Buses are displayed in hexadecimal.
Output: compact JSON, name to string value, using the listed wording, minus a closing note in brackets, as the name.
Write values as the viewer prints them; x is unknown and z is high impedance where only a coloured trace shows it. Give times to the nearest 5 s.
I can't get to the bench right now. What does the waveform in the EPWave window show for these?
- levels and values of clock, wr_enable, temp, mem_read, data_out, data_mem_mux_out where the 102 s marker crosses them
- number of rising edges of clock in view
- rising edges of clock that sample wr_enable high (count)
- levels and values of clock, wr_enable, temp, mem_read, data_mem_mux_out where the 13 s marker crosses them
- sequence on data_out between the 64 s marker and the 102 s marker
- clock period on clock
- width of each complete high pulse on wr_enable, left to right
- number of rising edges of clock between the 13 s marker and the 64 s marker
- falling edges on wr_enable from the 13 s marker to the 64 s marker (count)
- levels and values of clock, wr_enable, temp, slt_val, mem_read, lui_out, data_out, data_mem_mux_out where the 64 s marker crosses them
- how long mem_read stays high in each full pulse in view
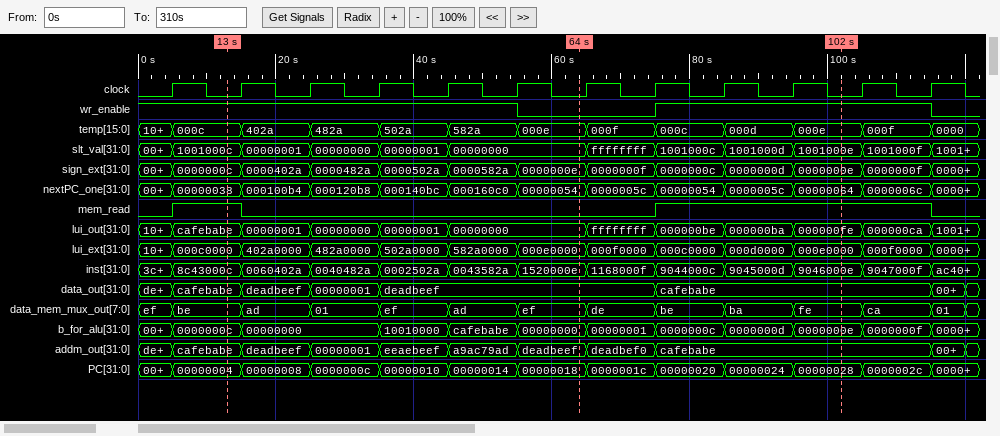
{"levels and values of clock, wr_enable, temp, mem_read, data_out, data_mem_mux_out where the 102 s marker crosses them": "clock=0, wr_enable=1, temp=000e, mem_read=1, data_out=cafebabe, data_mem_mux_out=fe", "number of rising edges of clock in view": "12", "rising edges of clock that sample wr_enable high": "10", "levels and values of clock, wr_enable, temp, mem_read, data_mem_mux_out where the 13 s marker crosses them": "clock=0, wr_enable=1, temp=000c, mem_read=1, data_mem_mux_out=be", "sequence on data_out between the 64 s marker and the 102 s marker": "deadbeef, cafebabe", "clock period on clock": "10 s", "width of each complete high pulse on wr_enable, left to right": "40 s", "number of rising edges of clock between the 13 s marker and the 64 s marker": "5", "falling edges on wr_enable from the 13 s marker to the 64 s marker": "1", "levels and values of clock, wr_enable, temp, slt_val, mem_read, lui_out, data_out, data_mem_mux_out where the 64 s marker crosses them": "clock=0, wr_enable=0, temp=000e, slt_val=00000000, mem_read=0, lui_out=00000000, data_out=deadbeef, data_mem_mux_out=ef", "how long mem_read stays high in each full pulse in view": "10 s, 40 s"}
